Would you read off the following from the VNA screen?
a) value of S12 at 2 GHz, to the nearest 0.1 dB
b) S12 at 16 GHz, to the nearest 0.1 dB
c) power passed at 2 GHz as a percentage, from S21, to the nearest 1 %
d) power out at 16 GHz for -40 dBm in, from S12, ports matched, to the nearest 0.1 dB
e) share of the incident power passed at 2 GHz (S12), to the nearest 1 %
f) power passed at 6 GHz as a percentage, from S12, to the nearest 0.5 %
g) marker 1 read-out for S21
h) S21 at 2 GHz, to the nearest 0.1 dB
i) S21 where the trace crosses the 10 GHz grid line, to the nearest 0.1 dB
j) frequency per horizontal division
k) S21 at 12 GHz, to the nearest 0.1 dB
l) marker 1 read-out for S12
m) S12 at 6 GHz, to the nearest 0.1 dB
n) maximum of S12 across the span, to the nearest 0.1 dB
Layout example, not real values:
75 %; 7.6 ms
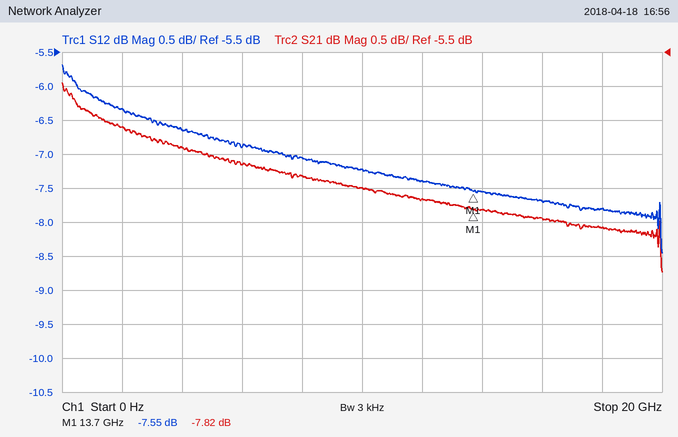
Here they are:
-6.3 dB; -7.7 dB; 22 %; -47.7 dBm; 23 %; 20.5 %; -7.82 dB; -6.6 dB; -7.5 dB; 2 GHz; -7.7 dB; -7.55 dB; -6.9 dB; -5.7 dB
